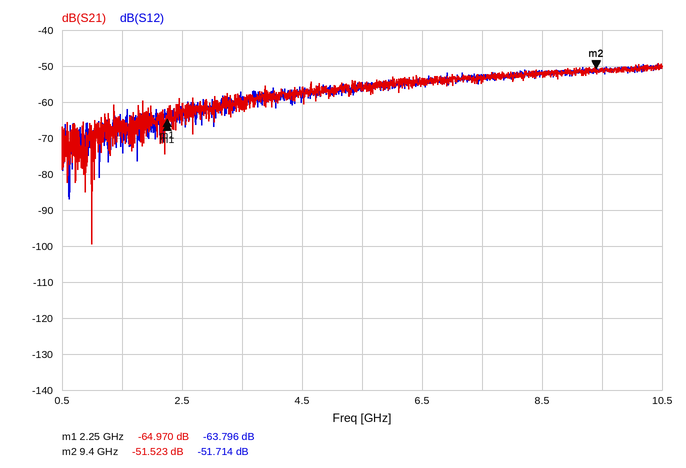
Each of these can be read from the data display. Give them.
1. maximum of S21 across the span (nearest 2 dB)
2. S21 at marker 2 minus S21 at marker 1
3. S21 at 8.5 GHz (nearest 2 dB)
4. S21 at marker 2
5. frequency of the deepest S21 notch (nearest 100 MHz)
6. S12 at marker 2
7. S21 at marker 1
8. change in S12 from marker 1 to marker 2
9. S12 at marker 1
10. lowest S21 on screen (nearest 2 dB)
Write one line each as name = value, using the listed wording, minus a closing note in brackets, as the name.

maximum of S21 across the span = -50 dB
S21 at marker 2 minus S21 at marker 1 = 13.447 dB
S21 at 8.5 GHz = -52 dB
S21 at marker 2 = -51.523 dB
frequency of the deepest S21 notch = 1.0 GHz
S12 at marker 2 = -51.714 dB
S21 at marker 1 = -64.970 dB
change in S12 from marker 1 to marker 2 = 12.082 dB
S12 at marker 1 = -63.796 dB
lowest S21 on screen = -100 dB
